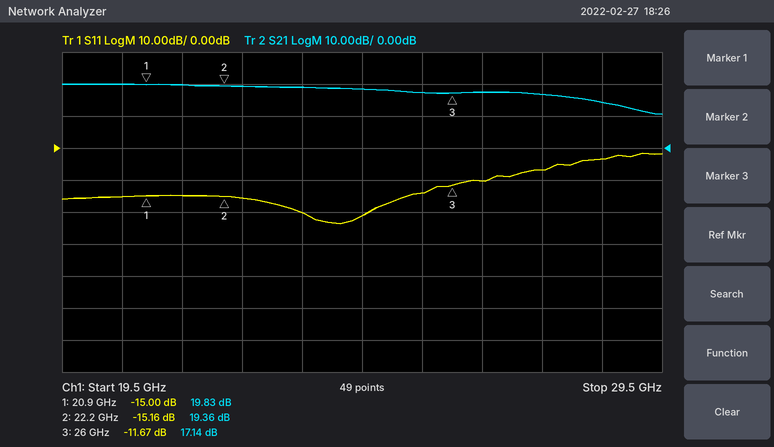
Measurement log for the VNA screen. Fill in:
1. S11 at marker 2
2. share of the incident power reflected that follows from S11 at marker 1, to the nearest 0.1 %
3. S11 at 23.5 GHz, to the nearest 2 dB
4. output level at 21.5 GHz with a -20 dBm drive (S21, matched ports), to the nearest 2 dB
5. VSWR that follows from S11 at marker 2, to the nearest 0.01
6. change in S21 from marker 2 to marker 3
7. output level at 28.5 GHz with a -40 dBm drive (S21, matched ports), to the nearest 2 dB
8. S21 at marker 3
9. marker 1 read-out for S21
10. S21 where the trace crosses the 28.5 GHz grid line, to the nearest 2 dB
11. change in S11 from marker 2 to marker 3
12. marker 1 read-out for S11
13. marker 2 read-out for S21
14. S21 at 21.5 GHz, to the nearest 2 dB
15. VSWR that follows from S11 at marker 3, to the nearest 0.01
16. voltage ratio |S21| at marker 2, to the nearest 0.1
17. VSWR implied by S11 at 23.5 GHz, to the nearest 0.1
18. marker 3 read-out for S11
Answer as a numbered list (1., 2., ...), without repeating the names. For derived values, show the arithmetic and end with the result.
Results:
1. -15.16 dB
2. 10^(-15/10) ≈ 3.2 %
3. -20 dB
4. -20 dBm + (20 dB) = 0 dBm
5. (1 + 0.1746)/(1 − 0.1746) ≈ 1.42
6. 17.14 − (19.36) = -2.22 dB
7. -40 dBm + (14 dB) = -26 dBm
8. 17.14 dB
9. 19.83 dB
10. 14 dB
11. -11.67 − (-15.16) = 3.49 dB
12. -15.00 dB
13. 19.36 dB
14. 20 dB
15. (1 + 0.2609)/(1 − 0.2609) ≈ 1.71
16. 10^(19.36/20) ≈ 9.3
17. |Γ| = 10^(-20/20) = 0.1000; VSWR = (1 + 0.1000)/(1 − 0.1000) ≈ 1.2
18. -11.67 dB
